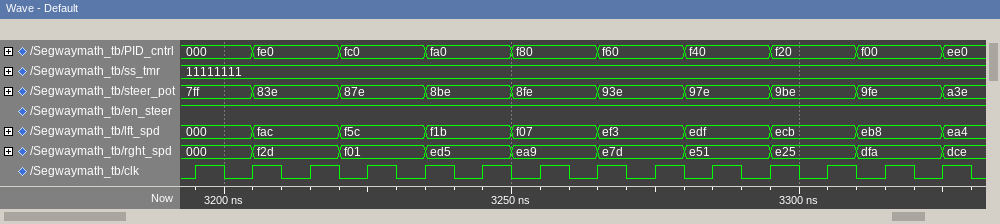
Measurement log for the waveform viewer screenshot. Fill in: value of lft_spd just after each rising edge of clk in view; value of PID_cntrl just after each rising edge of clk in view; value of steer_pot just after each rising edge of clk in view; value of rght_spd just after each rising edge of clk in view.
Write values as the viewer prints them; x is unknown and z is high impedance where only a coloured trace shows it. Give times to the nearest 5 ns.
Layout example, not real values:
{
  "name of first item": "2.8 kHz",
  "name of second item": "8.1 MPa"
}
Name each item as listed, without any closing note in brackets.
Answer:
{
  "value of lft_spd just after each rising edge of clk in view": "000, fac, fac, f5c, f1b, f1b, f07, ef3, ef3, edf, ecb, ecb, eb8, ea4",
  "value of PID_cntrl just after each rising edge of clk in view": "000, fe0, fe0, fc0, fa0, fa0, f80, f60, f60, f40, f20, f20, f00, ee0",
  "value of steer_pot just after each rising edge of clk in view": "7ff, 83e, 83e, 87e, 8be, 8be, 8fe, 93e, 93e, 97e, 9be, 9be, 9fe, a3e",
  "value of rght_spd just after each rising edge of clk in view": "000, f2d, f2d, f01, ed5, ed5, ea9, e7d, e7d, e51, e25, e25, dfa, dce"
}
